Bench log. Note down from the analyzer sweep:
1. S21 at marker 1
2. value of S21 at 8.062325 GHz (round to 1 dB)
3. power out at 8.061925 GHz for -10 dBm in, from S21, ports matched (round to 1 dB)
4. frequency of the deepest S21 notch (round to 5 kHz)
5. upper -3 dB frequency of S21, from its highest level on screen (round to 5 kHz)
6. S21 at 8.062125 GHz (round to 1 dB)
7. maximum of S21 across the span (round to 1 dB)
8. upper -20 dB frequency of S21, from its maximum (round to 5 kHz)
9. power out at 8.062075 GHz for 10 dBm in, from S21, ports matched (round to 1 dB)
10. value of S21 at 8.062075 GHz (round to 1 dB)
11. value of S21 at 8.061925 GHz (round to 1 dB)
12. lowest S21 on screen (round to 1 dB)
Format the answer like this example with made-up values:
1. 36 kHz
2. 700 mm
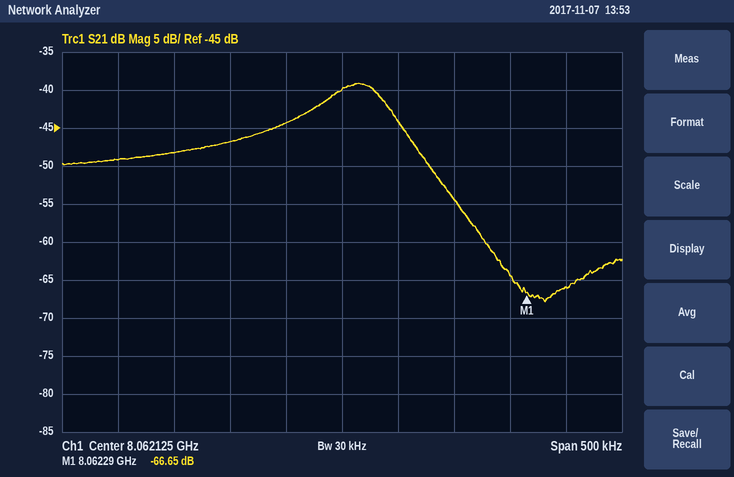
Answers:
1. -66.65 dB
2. -66 dB
3. -59 dBm
4. 8.062305 GHz
5. 8.062165 GHz
6. -40 dB
7. -39 dB
8. 8.062250 GHz
9. -34 dBm
10. -44 dB
11. -49 dB
12. -68 dB
